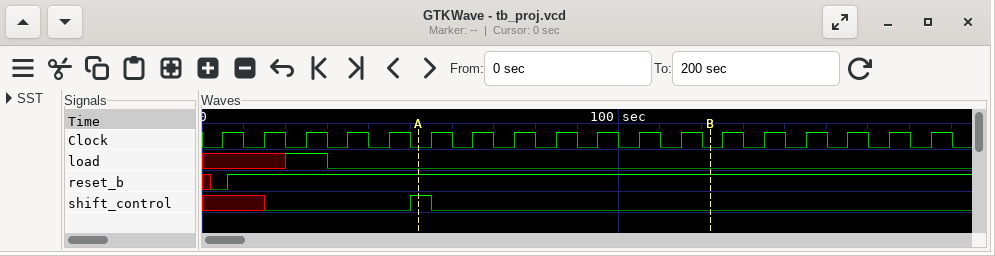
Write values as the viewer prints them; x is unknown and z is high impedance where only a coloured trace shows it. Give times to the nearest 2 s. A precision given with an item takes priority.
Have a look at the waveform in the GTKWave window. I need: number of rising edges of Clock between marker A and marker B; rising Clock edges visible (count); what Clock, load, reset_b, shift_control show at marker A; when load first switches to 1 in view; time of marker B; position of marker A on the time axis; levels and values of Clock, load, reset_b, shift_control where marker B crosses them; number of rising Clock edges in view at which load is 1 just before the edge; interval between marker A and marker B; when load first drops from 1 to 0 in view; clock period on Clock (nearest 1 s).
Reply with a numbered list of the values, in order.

1. 7
2. 18
3. Clock=0, load=0, reset_b=1, shift_control=1
4. 20 s
5. 122 s
6. 52 s
7. Clock=0, load=0, reset_b=1, shift_control=0
8. 1
9. 70 s
10. 30 s
11. 10 s
